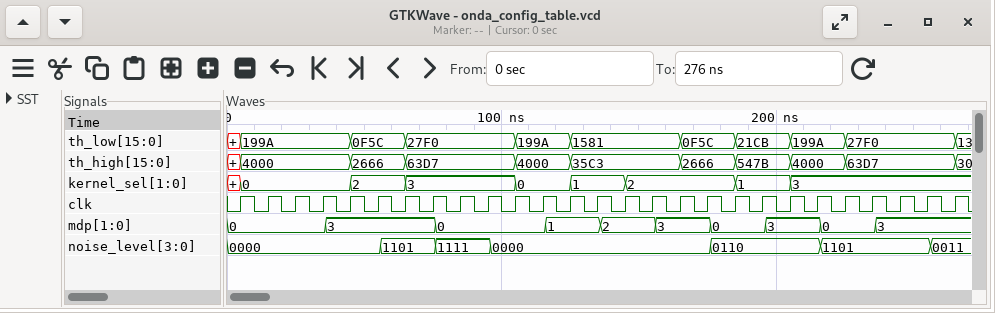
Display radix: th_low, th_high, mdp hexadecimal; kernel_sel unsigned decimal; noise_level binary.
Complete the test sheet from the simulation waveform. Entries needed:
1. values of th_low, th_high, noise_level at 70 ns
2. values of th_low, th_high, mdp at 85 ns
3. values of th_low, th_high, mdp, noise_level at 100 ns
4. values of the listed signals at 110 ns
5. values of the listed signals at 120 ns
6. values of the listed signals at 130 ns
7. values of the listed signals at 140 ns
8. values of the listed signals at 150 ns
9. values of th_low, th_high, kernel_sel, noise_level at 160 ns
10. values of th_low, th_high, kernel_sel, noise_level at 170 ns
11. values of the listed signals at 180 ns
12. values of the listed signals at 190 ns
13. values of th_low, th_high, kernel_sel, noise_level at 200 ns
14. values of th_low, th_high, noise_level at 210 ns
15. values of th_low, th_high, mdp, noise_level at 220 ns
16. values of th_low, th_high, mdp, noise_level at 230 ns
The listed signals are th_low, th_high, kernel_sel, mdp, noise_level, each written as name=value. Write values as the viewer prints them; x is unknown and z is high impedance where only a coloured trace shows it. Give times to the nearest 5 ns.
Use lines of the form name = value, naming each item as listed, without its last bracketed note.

values of th_low, th_high, noise_level at 70 ns = th_low=27F0, th_high=63D7, noise_level=1101
values of th_low, th_high, mdp at 85 ns = th_low=27F0, th_high=63D7, mdp=0
values of th_low, th_high, mdp, noise_level at 100 ns = th_low=27F0, th_high=63D7, mdp=0, noise_level=0000
values of the listed signals at 110 ns = th_low=199A, th_high=4000, kernel_sel=0, mdp=0, noise_level=0000
values of the listed signals at 120 ns = th_low=199A, th_high=4000, kernel_sel=0, mdp=1, noise_level=0000
values of the listed signals at 130 ns = th_low=1581, th_high=35C3, kernel_sel=1, mdp=1, noise_level=0000
values of the listed signals at 140 ns = th_low=1581, th_high=35C3, kernel_sel=1, mdp=2, noise_level=0000
values of the listed signals at 150 ns = th_low=1581, th_high=35C3, kernel_sel=2, mdp=2, noise_level=0000
values of th_low, th_high, kernel_sel, noise_level at 160 ns = th_low=1581, th_high=35C3, kernel_sel=2, noise_level=0000
values of th_low, th_high, kernel_sel, noise_level at 170 ns = th_low=0F5C, th_high=2666, kernel_sel=2, noise_level=0000
values of the listed signals at 180 ns = th_low=0F5C, th_high=2666, kernel_sel=2, mdp=0, noise_level=0110
values of the listed signals at 190 ns = th_low=21CB, th_high=547B, kernel_sel=1, mdp=0, noise_level=0110
values of th_low, th_high, kernel_sel, noise_level at 200 ns = th_low=21CB, th_high=547B, kernel_sel=1, noise_level=0110
values of th_low, th_high, noise_level at 210 ns = th_low=199A, th_high=4000, noise_level=0110
values of th_low, th_high, mdp, noise_level at 220 ns = th_low=199A, th_high=4000, mdp=0, noise_level=1101
values of th_low, th_high, mdp, noise_level at 230 ns = th_low=27F0, th_high=63D7, mdp=0, noise_level=1101
